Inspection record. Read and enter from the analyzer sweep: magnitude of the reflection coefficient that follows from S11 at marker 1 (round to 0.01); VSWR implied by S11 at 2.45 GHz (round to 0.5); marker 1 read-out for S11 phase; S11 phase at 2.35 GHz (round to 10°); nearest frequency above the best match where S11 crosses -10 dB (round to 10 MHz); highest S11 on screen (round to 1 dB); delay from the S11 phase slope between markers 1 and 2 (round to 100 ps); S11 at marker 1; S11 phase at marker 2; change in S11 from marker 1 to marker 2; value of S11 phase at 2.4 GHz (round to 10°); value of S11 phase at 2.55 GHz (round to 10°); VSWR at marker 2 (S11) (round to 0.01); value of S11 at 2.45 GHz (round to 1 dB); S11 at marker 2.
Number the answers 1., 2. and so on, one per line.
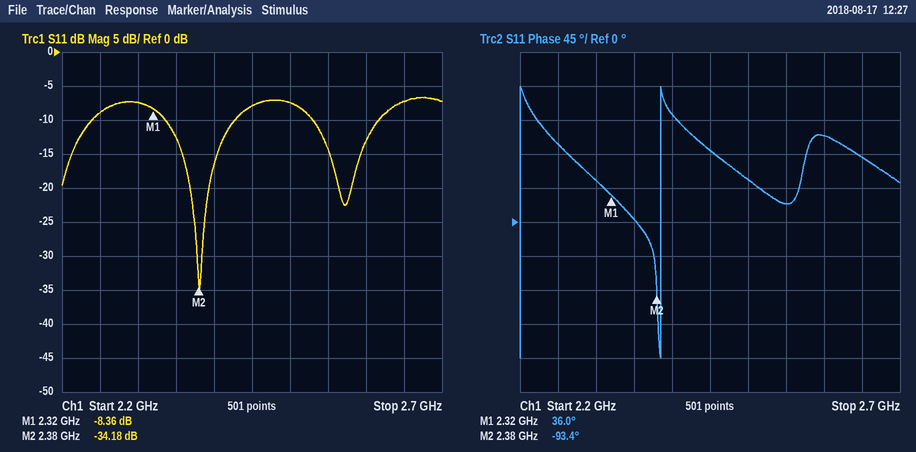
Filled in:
1. 0.38
2. 2.5
3. 36.0°
4. 0°
5. 2.43 GHz
6. -7 dB
7. 6.0 ns
8. -8.36 dB
9. -93.4°
10. -25.82 dB
11. 140°
12. 20°
13. 1.04
14. -8 dB
15. -34.18 dB
